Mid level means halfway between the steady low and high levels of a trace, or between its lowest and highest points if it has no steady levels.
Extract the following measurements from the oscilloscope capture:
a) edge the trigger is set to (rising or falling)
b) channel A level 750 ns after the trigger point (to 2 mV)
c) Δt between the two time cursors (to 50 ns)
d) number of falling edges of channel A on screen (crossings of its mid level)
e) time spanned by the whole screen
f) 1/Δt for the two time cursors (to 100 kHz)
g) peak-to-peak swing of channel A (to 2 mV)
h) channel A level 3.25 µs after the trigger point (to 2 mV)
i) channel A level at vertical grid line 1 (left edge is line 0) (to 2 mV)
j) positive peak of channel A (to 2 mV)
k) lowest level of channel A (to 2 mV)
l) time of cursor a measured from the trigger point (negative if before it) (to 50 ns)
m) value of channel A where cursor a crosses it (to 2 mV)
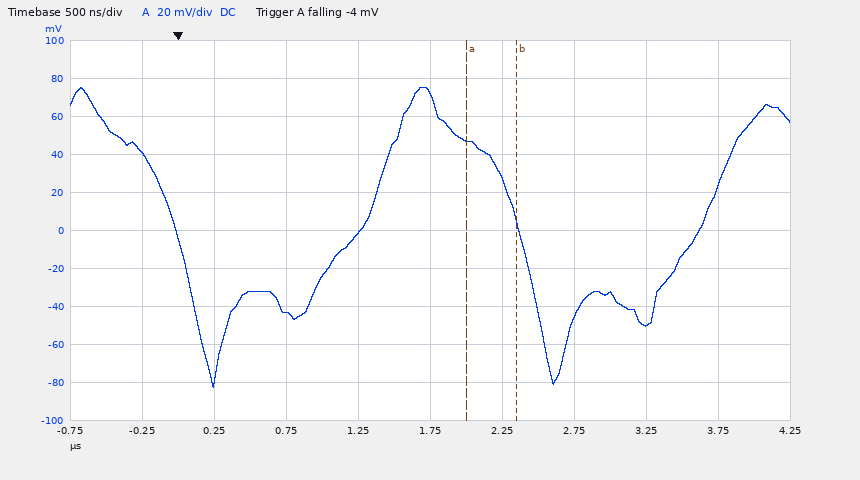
falling
-44 mV
350 ns
2
5 µs
2.9 MHz
158 mV
-50 mV
40 mV
76 mV
-82 mV
+2.00 µs
48 mV
